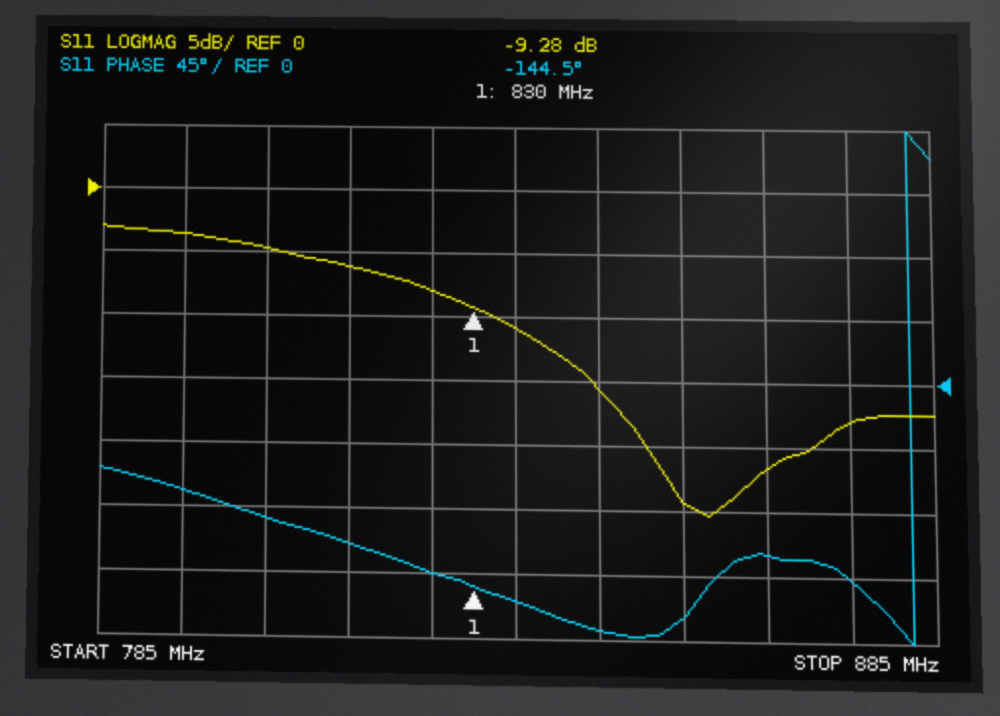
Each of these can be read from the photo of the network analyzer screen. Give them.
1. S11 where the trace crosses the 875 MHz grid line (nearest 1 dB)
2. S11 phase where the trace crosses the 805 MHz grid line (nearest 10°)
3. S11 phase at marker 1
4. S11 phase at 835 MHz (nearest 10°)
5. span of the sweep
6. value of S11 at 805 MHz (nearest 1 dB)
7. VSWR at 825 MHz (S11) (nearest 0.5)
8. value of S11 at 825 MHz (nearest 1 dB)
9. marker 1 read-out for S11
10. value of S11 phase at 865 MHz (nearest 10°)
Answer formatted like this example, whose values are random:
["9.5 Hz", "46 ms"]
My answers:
["-18 dB", "-100°", "-144.5°", "-150°", "100 MHz", "-5 dB", "2.5", "-8 dB", "-9.28 dB", "-120°"]
